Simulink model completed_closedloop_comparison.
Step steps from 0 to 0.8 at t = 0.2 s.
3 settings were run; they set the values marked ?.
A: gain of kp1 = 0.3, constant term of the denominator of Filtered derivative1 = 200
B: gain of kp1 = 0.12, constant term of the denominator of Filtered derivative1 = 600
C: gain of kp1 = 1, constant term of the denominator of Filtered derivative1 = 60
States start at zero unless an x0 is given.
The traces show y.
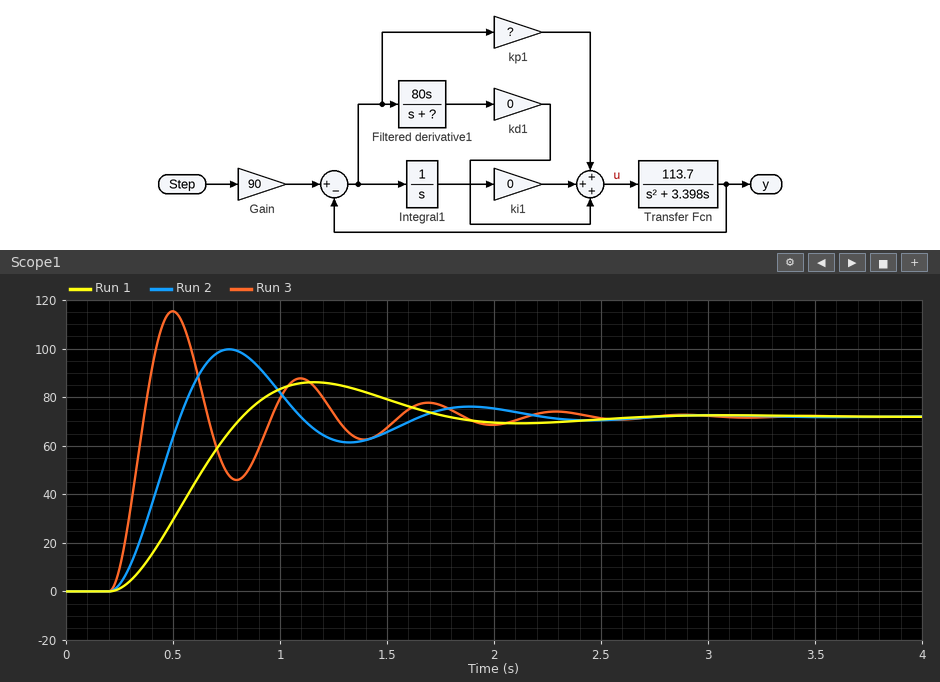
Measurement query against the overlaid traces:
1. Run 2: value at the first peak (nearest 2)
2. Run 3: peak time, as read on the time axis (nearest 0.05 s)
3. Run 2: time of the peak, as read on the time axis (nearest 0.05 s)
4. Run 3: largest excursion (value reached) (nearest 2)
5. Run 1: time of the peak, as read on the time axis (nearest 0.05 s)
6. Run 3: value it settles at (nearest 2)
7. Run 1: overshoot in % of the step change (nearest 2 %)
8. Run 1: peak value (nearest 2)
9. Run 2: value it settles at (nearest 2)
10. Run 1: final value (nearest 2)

100
0.50 s
0.75 s
116
1.15 s
72
20 %
86
72
72
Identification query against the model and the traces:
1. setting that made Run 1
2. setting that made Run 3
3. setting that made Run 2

B
C
A
